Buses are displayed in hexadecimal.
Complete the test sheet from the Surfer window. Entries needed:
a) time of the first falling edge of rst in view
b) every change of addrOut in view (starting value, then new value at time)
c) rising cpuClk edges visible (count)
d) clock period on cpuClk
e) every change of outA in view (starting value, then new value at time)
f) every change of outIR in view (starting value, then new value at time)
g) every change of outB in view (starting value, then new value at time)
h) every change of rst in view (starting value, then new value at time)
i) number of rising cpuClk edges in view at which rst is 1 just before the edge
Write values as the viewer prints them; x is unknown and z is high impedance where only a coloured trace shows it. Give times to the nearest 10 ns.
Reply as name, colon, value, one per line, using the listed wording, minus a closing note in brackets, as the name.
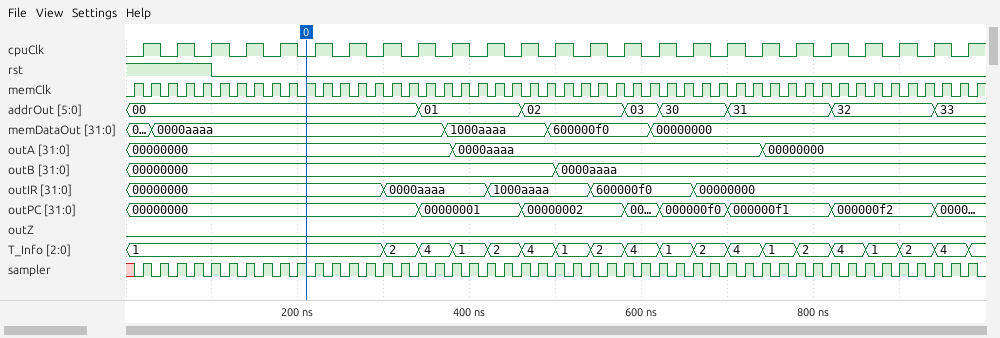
time of the first falling edge of rst in view: 100 ns
every change of addrOut in view: 00, 01 at 340 ns, 02 at 460 ns, 03 at 580 ns, 30 at 620 ns, 31 at 700 ns, 32 at 820 ns, 33 at 940 ns
rising cpuClk edges visible: 25
clock period on cpuClk: 40 ns
every change of outA in view: 00000000, 0000aaaa at 380 ns, 00000000 at 740 ns
every change of outIR in view: 00000000, 0000aaaa at 300 ns, 1000aaaa at 420 ns, 600000f0 at 540 ns, 00000000 at 660 ns
every change of outB in view: 00000000, 0000aaaa at 500 ns
every change of rst in view: 1, 0 at 100 ns
number of rising cpuClk edges in view at which rst is 1 just before the edge: 3
